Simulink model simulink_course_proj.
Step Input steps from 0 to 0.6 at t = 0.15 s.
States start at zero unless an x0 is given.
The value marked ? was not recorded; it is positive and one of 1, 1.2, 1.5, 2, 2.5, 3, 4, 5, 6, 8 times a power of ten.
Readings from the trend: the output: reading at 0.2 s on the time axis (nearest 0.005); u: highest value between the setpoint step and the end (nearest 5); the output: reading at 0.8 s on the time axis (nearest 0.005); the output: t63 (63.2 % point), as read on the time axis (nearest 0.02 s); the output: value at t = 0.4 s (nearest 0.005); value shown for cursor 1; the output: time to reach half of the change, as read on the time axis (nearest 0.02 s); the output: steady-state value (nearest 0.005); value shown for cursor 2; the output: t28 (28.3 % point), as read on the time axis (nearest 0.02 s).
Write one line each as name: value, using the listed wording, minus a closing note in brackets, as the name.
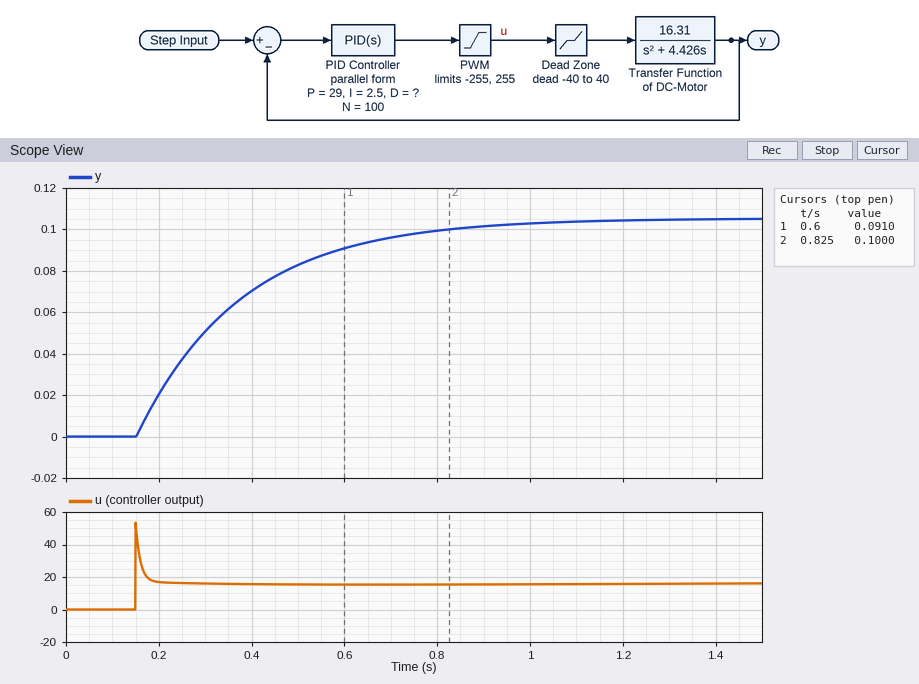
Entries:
the output: reading at 0.2 s on the time axis: 0.020
u: highest value between the setpoint step and the end: 55
the output: reading at 0.8 s on the time axis: 0.100
the output: t63 (63.2 % point), as read on the time axis: 0.38 s
the output: value at t = 0.4 s: 0.070
value shown for cursor 1: 0.0910
the output: time to reach half of the change, as read on the time axis: 0.30 s
the output: steady-state value: 0.105
value shown for cursor 2: 0.1000
the output: t28 (28.3 % point), as read on the time axis: 0.22 s
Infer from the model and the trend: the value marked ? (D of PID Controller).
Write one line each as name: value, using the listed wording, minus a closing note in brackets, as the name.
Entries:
the value marked ?: 0.6
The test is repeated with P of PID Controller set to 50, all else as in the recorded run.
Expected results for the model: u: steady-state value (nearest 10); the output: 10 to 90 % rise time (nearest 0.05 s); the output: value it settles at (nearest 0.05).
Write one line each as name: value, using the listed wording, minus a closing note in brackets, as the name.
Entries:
u: steady-state value: 10
the output: 10 to 90 % rise time: 0.50 s
the output: value it settles at: 0.45
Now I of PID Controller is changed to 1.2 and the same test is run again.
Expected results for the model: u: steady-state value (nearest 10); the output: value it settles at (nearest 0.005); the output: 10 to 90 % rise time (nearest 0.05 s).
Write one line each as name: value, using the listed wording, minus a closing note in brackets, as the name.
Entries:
u: steady-state value: 20
the output: value it settles at: 0.105
the output: 10 to 90 % rise time: 0.50 s
